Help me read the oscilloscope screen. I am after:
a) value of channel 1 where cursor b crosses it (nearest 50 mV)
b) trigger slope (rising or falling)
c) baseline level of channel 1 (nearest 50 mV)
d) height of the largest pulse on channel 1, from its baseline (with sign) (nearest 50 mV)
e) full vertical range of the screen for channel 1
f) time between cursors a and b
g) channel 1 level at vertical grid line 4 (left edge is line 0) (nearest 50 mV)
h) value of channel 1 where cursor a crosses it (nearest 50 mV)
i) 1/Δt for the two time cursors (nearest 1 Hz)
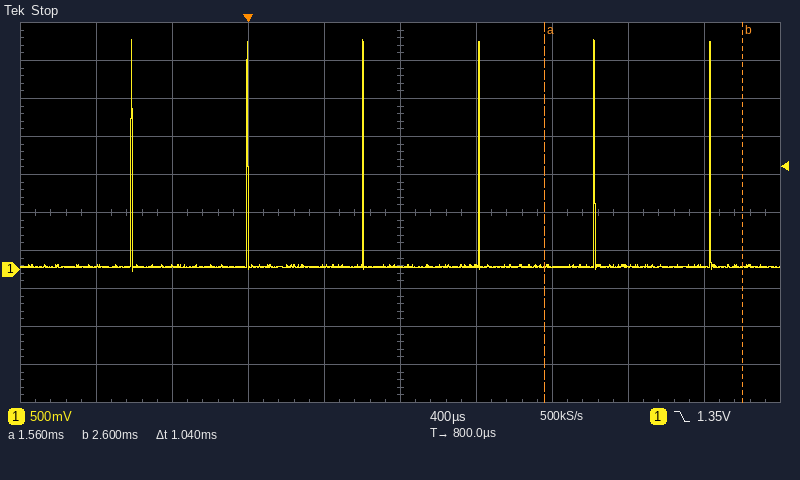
50 mV
falling
50 mV
+3.00 V
5 V
1.04 ms
50 mV
50 mV
962 Hz
